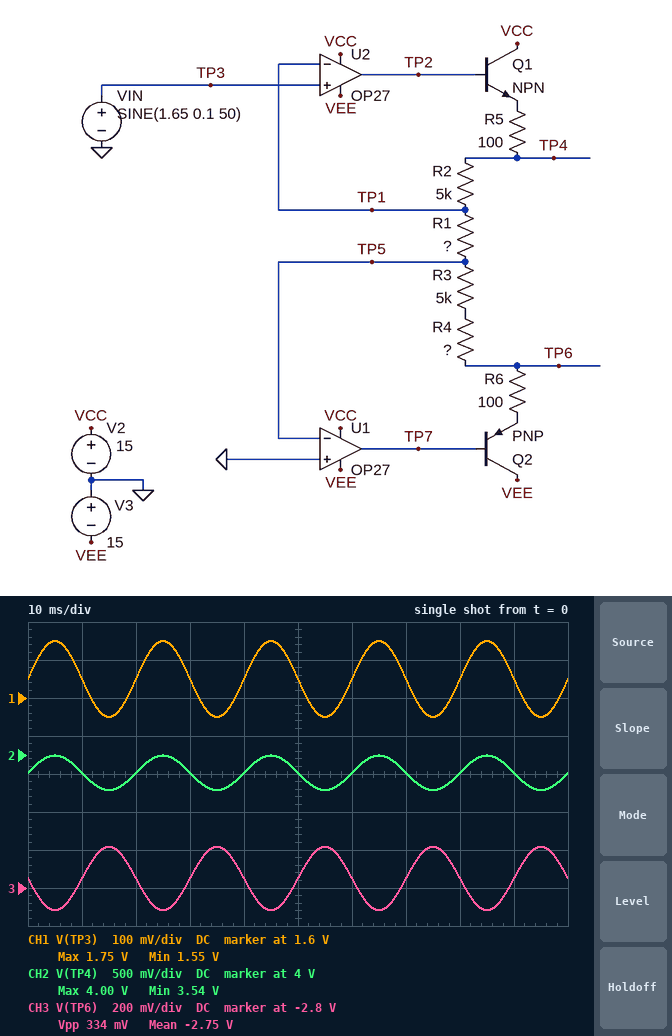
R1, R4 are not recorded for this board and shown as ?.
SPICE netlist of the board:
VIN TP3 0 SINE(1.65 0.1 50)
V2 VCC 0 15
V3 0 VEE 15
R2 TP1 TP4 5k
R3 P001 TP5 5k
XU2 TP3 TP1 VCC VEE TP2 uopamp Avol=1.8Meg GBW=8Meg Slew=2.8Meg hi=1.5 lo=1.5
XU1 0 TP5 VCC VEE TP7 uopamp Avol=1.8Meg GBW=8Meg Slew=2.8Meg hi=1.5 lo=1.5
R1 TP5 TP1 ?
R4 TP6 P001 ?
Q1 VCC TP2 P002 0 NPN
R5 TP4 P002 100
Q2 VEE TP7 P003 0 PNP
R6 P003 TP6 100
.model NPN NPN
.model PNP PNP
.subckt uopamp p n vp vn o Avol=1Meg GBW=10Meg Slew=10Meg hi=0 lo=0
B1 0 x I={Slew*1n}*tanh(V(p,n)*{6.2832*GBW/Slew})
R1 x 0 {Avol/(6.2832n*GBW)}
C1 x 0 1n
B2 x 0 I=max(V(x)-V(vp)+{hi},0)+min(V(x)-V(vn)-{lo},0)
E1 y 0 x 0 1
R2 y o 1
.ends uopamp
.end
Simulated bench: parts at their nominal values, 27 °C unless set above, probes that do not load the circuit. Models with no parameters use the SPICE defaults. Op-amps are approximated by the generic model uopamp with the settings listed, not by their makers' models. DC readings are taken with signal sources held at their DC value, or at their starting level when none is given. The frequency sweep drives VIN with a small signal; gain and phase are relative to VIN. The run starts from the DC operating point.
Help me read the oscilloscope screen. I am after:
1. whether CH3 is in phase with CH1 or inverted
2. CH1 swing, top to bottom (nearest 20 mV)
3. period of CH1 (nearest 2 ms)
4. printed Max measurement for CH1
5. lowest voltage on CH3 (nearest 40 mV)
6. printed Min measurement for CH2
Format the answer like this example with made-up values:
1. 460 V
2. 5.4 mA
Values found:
1. inverted
2. 200 mV
3. 20 ms
4. 1.75 V
5. -2.92 V
6. 3.54 V
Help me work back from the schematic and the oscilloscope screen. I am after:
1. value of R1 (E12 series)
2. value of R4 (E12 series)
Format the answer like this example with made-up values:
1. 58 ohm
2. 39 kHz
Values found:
1. 3.9 kΩ
2. 1.5 kΩ
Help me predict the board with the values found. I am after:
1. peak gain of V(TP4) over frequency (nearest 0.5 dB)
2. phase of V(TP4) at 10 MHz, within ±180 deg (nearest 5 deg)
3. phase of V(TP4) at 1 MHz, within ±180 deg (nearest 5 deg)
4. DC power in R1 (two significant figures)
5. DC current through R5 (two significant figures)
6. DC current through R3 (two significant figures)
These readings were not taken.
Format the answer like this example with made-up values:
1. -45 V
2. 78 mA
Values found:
1. 7.0 dB
2. -65 deg
3. -20 deg
4. 700 µW
5. 420 µA
6. 420 µA
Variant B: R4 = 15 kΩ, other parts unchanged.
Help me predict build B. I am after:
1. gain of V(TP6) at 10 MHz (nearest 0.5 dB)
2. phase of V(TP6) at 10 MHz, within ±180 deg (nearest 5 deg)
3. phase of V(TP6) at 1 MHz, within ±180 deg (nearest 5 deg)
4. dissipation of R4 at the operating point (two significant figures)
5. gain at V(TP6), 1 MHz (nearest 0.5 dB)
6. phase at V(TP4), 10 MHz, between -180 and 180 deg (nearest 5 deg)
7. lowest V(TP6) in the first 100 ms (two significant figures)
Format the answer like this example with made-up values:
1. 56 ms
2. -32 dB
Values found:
1. -9.5 dB
2. 45 deg
3. 130 deg
4. 2.7 mW
5. 11.5 dB
6. -60 deg
7. -9.0 V
